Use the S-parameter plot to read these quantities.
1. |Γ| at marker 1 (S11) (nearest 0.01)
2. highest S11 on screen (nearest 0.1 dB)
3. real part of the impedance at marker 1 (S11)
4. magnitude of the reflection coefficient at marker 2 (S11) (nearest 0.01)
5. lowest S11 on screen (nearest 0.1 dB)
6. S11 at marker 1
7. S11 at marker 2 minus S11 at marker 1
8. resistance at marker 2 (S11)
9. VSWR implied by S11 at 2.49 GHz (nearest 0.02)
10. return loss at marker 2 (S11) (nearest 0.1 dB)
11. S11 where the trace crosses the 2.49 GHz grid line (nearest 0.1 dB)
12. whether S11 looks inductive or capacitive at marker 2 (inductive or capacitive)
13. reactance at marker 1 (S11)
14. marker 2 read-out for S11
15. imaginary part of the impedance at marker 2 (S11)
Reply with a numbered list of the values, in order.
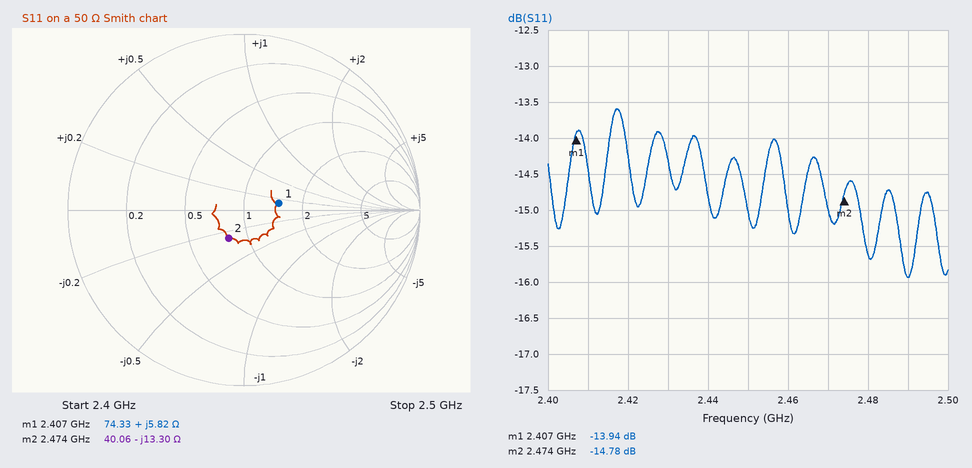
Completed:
1. 0.20
2. -13.6 dB
3. 74.33 Ω
4. 0.18
5. -15.9 dB
6. -13.94 dB
7. -0.84 dB
8. 40.06 Ω
9. 1.38
10. 14.8 dB
11. -15.9 dB
12. capacitive
13. +5.82 Ω
14. -14.78 dB
15. -13.30 Ω
